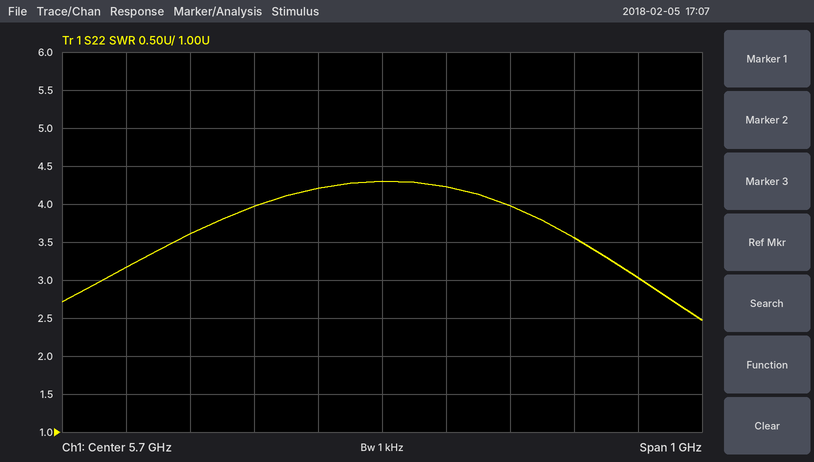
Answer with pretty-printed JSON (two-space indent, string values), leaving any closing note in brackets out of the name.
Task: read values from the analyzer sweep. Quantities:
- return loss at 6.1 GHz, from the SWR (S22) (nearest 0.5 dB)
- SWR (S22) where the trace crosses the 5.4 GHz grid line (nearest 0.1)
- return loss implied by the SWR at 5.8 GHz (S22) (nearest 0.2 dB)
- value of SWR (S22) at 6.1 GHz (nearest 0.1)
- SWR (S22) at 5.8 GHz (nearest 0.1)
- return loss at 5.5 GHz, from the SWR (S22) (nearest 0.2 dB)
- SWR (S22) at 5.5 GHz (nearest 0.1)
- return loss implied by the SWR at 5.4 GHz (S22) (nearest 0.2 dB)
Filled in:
{
  "return loss at 6.1 GHz, from the SWR (S22)": "6.0 dB",
  "SWR (S22) where the trace crosses the 5.4 GHz grid line": "3.6",
  "return loss implied by the SWR at 5.8 GHz (S22)": "4.2 dB",
  "value of SWR (S22) at 6.1 GHz": "3.0",
  "SWR (S22) at 5.8 GHz": "4.2",
  "return loss at 5.5 GHz, from the SWR (S22)": "4.4 dB",
  "SWR (S22) at 5.5 GHz": "4.0",
  "return loss implied by the SWR at 5.4 GHz (S22)": "5.0 dB"
}
